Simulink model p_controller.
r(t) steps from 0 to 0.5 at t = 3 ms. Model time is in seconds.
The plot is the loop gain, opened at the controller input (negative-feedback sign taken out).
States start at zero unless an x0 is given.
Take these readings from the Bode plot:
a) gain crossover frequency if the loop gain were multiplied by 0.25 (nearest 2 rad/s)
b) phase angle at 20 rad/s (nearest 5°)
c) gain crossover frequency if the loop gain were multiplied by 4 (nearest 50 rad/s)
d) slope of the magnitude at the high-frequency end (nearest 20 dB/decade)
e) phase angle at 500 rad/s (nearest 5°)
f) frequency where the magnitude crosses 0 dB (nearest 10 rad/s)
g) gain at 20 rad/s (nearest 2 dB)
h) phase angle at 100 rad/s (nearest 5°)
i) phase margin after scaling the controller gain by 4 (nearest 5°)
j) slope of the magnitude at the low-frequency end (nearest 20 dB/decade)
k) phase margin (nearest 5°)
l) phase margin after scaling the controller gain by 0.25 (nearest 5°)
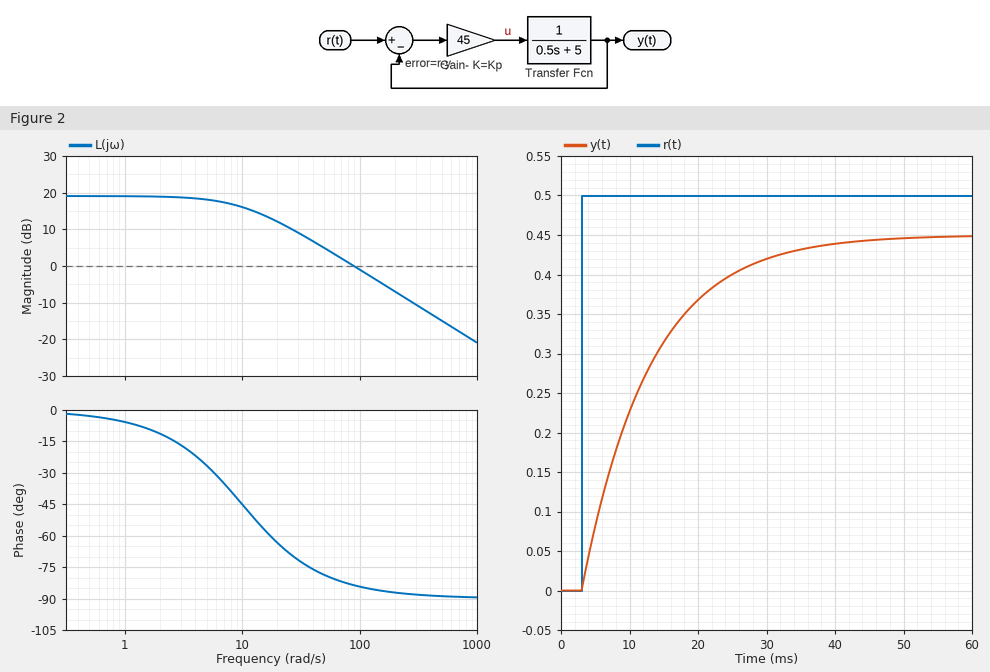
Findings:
20 rad/s
-65°
350 rad/s
-20 dB/decade
-90°
90 rad/s
12 dB
-85°
90°
0 dB/decade
95°
115°
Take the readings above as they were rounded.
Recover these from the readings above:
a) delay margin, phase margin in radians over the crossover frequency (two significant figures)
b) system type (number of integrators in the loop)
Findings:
0.018 s
0
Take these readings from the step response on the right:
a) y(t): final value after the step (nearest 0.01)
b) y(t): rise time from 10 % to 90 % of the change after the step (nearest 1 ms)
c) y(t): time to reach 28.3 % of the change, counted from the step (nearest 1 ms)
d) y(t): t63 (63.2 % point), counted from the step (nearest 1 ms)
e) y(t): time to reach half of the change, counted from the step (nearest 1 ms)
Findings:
0.45
22 ms
3 ms
10 ms
7 ms
